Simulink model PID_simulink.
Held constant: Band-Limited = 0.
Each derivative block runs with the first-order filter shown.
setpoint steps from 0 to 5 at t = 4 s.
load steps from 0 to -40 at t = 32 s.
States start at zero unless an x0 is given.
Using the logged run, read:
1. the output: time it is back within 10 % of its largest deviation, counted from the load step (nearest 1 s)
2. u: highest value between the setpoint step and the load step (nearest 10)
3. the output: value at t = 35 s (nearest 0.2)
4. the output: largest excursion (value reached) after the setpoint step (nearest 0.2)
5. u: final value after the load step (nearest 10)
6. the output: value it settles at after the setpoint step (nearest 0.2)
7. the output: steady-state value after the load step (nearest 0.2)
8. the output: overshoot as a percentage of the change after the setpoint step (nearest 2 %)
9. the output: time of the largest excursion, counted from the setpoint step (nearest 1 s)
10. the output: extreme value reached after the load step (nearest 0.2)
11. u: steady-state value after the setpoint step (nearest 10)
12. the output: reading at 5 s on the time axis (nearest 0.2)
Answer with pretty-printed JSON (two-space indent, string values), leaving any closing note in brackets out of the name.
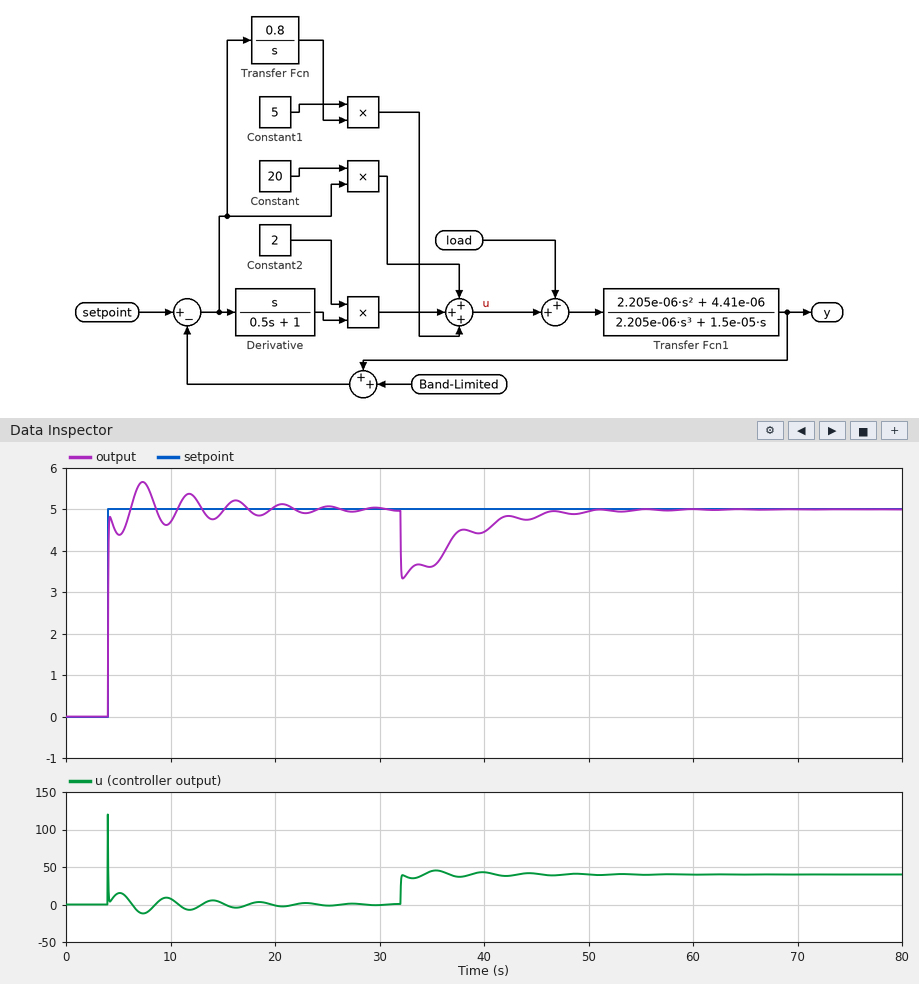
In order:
{
  "the output: time it is back within 10 % of its largest deviation, counted from the load step": "13 s",
  "u: highest value between the setpoint step and the load step": "120",
  "the output: value at t = 35 s": "3.6",
  "the output: largest excursion (value reached) after the setpoint step": "5.6",
  "u: final value after the load step": "40",
  "the output: value it settles at after the setpoint step": "5.0",
  "the output: steady-state value after the load step": "5.0",
  "the output: overshoot as a percentage of the change after the setpoint step": "14 %",
  "the output: time of the largest excursion, counted from the setpoint step": "3 s",
  "the output: extreme value reached after the load step": "3.4",
  "u: steady-state value after the setpoint step": "0",
  "the output: reading at 5 s on the time axis": "4.4"
}
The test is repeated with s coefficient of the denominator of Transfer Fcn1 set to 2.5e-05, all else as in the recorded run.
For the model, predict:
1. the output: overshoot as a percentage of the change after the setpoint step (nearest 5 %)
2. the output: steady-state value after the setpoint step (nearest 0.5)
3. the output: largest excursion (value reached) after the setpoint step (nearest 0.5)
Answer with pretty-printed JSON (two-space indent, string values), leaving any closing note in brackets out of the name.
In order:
{
  "the output: overshoot as a percentage of the change after the setpoint step": "20 %",
  "the output: steady-state value after the setpoint step": "5.0",
  "the output: largest excursion (value reached) after the setpoint step": "6.0"
}
